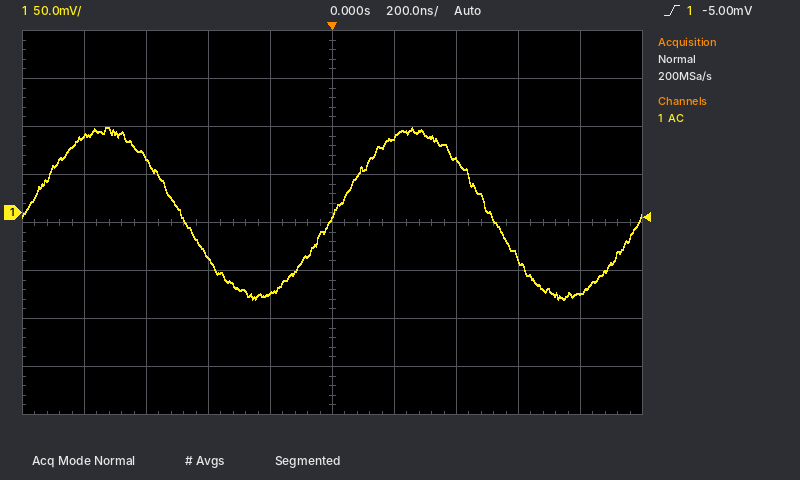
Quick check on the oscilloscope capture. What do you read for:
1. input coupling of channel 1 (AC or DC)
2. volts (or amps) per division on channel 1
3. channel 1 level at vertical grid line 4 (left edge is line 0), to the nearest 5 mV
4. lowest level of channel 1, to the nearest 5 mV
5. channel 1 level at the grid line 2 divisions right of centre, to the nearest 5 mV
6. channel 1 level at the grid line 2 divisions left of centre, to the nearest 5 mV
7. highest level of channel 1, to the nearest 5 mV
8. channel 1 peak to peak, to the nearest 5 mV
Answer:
AC
50 mV
-85 mV
-90 mV
55 mV
-45 mV
90 mV
180 mV
